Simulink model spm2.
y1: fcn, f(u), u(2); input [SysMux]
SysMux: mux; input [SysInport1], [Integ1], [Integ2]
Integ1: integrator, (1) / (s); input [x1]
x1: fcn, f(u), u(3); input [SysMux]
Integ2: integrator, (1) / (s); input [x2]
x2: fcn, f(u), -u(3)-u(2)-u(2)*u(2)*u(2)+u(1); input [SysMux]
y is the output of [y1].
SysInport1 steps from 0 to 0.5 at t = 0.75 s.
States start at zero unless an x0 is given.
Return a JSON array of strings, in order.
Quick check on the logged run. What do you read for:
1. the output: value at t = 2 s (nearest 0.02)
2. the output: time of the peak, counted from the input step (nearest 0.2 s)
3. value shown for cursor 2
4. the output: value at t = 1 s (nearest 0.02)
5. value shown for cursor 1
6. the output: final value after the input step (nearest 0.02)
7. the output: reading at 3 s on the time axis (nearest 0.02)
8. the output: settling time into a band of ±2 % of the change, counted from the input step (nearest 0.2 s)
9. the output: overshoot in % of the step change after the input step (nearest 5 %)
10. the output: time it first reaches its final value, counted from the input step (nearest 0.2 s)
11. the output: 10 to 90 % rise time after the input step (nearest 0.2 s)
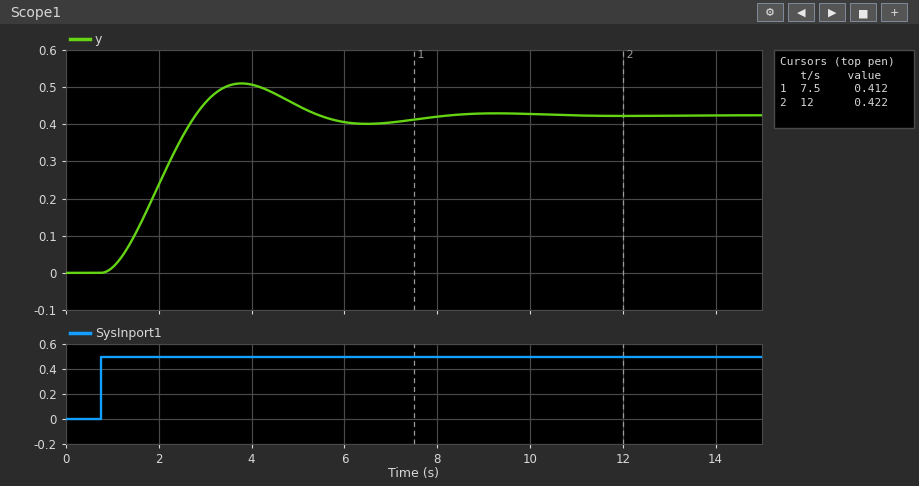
["0.24", "3.0 s", "0.422", "0.02", "0.412", "0.42", "0.46", "7.0 s", "20 %", "2.0 s", "1.4 s"]
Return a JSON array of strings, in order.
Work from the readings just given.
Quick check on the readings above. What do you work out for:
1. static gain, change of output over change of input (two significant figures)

["0.84"]
